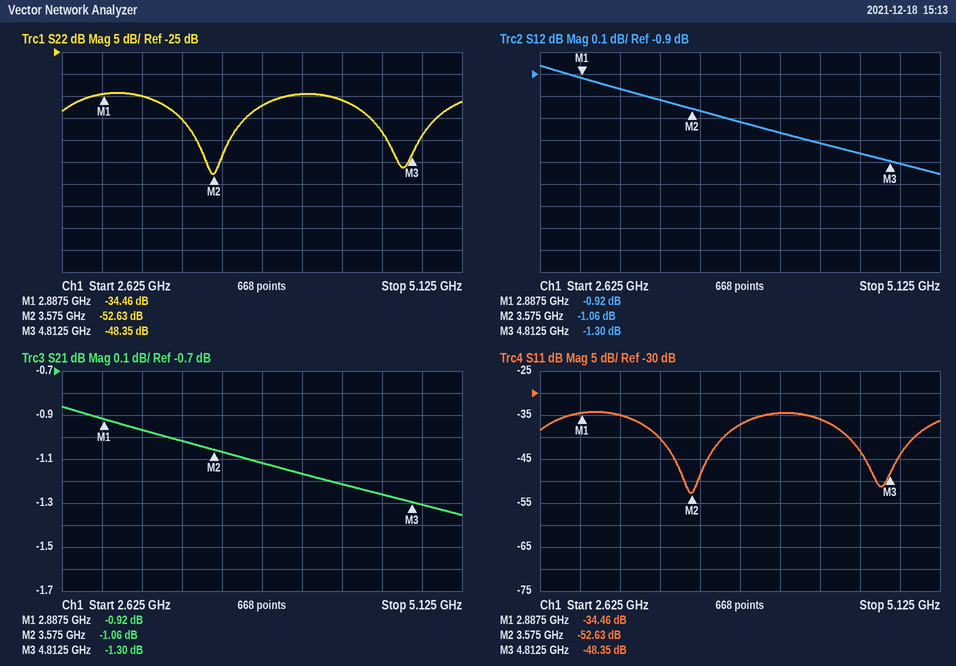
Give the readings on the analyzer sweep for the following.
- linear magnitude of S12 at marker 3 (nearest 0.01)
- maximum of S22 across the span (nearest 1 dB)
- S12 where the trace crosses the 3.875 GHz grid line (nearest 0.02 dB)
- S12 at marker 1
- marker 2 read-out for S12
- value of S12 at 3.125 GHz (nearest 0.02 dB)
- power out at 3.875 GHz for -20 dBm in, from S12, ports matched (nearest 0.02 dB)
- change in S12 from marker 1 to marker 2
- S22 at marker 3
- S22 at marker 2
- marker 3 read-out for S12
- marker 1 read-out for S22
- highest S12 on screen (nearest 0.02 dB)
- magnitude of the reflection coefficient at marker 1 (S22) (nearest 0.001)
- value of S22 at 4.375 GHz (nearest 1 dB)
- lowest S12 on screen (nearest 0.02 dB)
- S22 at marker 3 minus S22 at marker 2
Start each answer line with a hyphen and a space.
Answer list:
- 0.86
- -34 dB
- -1.12 dB
- -0.92 dB
- -1.06 dB
- -0.96 dB
- -21.12 dBm
- -0.14 dB
- -48.35 dB
- -52.63 dB
- -1.30 dB
- -34.46 dB
- -0.86 dB
- 0.019
- -36 dB
- -1.36 dB
- 4.28 dB
